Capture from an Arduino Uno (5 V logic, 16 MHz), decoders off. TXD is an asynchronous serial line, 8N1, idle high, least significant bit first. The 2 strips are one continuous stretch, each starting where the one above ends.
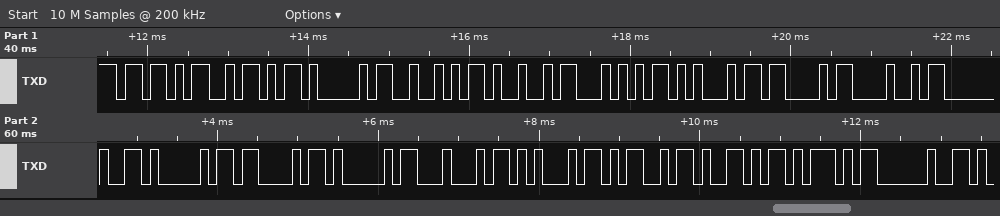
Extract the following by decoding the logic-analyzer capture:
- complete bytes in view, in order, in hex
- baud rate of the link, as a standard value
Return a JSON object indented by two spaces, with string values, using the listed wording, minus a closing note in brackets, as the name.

{
  "complete bytes in view, in order, in hex": "5B 5A 41 52 49 54 45 43 48 20 41 43 41 44 45 4D 59 5D 20",
  "baud rate of the link, as a standard value": "9600 baud"
}
